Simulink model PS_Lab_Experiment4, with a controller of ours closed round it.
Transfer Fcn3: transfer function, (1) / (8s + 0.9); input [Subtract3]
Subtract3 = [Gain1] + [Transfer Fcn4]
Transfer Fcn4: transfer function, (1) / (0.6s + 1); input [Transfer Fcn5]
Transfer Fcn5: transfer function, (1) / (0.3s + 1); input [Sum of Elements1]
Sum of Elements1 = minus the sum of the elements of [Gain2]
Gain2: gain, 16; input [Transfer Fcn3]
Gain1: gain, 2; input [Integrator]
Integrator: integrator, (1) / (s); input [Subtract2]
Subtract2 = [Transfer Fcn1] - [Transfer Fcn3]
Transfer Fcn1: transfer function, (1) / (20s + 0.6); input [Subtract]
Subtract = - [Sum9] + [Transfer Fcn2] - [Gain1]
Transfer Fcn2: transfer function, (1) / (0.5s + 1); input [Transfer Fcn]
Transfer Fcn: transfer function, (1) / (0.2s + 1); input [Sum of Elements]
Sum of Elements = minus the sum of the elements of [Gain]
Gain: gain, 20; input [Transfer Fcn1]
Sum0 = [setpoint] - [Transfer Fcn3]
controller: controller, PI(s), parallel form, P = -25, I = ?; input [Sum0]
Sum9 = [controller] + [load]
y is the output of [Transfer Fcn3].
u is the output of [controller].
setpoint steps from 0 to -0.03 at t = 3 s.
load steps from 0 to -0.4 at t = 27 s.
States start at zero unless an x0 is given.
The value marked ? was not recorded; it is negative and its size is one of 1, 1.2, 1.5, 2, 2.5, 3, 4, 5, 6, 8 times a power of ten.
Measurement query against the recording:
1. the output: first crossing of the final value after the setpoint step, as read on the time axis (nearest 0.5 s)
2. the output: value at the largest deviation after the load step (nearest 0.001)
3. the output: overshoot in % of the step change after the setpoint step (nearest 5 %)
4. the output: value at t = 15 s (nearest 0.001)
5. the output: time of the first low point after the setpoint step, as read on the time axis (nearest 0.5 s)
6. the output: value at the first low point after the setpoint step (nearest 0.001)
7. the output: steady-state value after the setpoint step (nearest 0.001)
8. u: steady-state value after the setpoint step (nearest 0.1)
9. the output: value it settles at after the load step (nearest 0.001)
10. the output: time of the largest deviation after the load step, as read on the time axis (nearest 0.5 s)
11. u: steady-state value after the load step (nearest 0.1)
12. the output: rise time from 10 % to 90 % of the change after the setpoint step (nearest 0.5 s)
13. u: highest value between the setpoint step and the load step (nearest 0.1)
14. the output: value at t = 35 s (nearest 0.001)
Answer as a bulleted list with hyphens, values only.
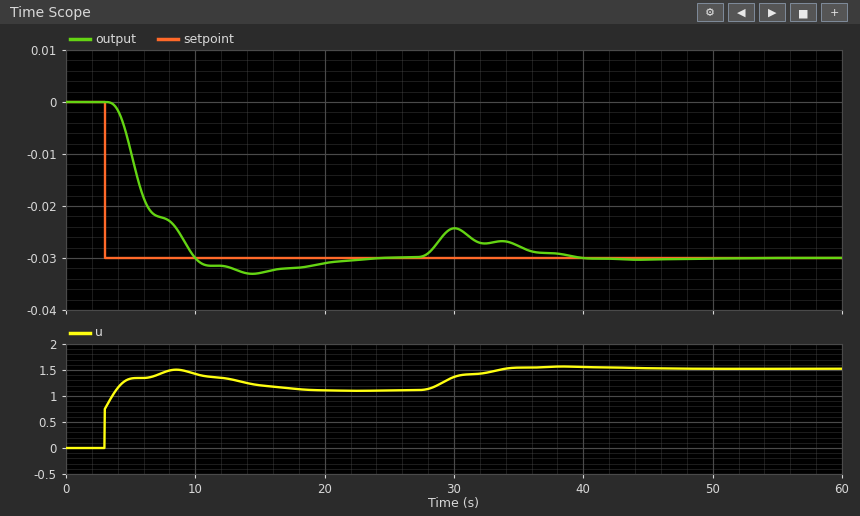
- 10.0 s
- -0.024
- 10 %
- -0.033
- 14.5 s
- -0.033
- -0.030
- 1.1
- -0.030
- 30.0 s
- 1.5
- 5.0 s
- 1.5
- -0.028
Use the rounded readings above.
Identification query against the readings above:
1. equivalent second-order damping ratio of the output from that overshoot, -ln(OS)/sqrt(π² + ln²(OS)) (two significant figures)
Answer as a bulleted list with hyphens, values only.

- 0.59
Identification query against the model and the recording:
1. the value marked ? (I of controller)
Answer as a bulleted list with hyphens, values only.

- -15
